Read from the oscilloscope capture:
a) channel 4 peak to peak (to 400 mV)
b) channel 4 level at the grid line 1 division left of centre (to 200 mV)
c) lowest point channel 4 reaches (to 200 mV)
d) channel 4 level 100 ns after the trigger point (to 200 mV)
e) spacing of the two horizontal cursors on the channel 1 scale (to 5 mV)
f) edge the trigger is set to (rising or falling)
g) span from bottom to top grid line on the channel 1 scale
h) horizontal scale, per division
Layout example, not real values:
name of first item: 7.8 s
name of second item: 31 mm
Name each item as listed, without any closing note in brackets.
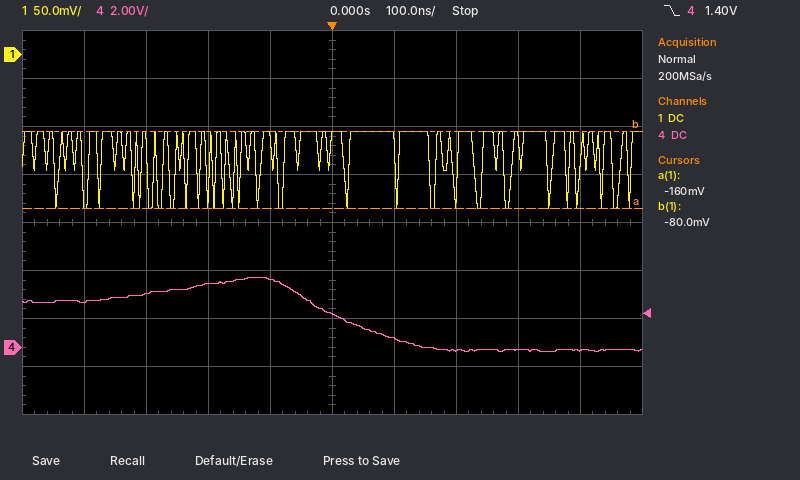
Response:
channel 4 peak to peak: 3.2 V
channel 4 level at the grid line 1 division left of centre: 2.8 V
lowest point channel 4 reaches: -200 mV
channel 4 level 100 ns after the trigger point: 400 mV
spacing of the two horizontal cursors on the channel 1 scale: 80 mV
edge the trigger is set to: falling
span from bottom to top grid line on the channel 1 scale: 400 mV
horizontal scale, per division: 100 ns
